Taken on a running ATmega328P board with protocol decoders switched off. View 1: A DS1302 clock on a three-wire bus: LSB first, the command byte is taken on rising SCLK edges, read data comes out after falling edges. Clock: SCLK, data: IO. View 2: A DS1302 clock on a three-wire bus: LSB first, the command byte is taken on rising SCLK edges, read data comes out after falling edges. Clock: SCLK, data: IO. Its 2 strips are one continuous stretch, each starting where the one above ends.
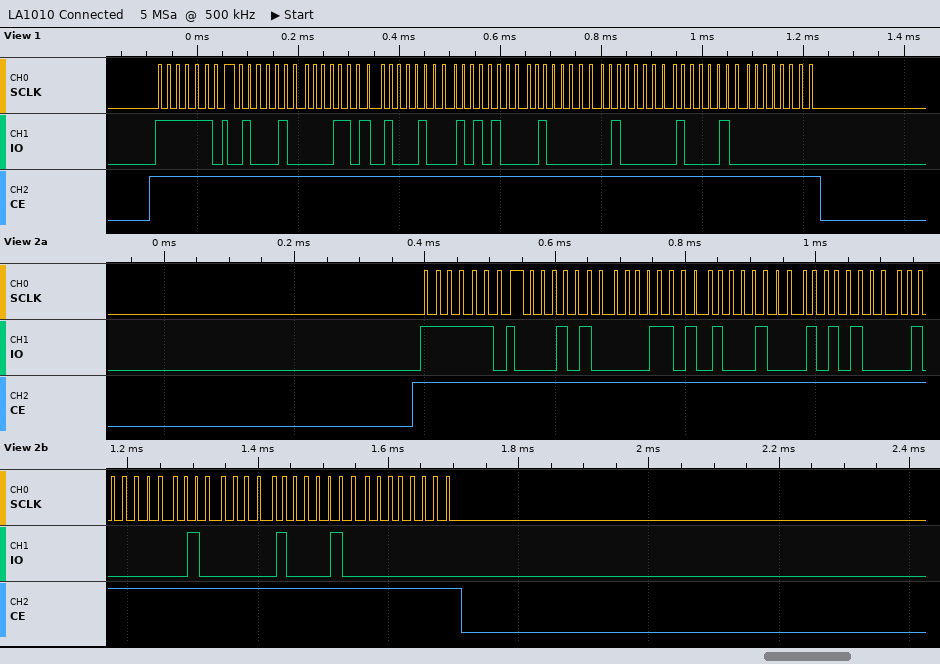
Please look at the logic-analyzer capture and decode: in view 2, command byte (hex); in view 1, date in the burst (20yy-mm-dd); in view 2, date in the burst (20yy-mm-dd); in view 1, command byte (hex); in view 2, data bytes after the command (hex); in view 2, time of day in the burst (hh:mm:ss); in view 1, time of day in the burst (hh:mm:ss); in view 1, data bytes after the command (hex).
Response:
0xBF
2021-02-15
2021-02-15
0xBF
28 58 11 15 02 02 21 00
11:58:28
11:58:22
22 58 11 15 02 02 21 00
